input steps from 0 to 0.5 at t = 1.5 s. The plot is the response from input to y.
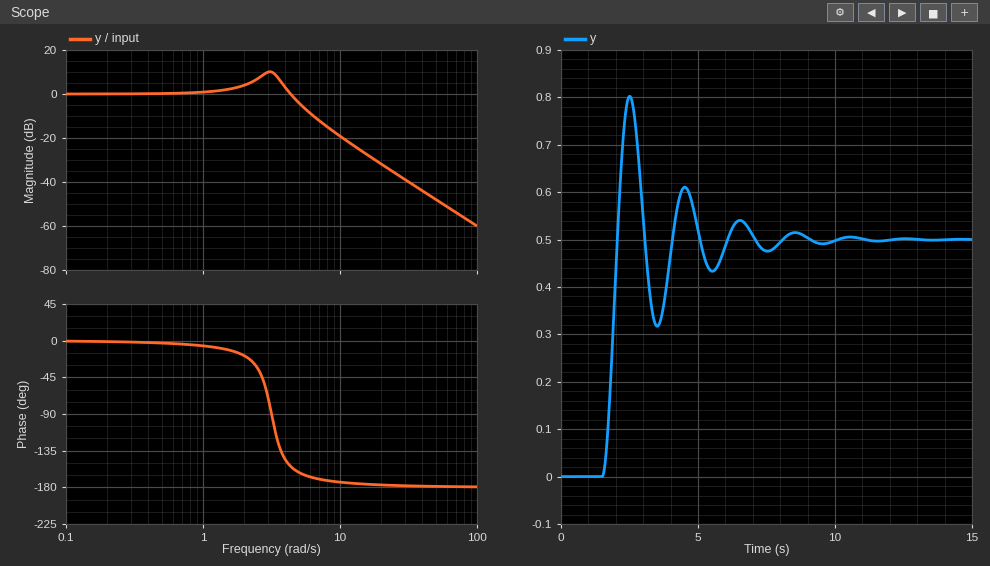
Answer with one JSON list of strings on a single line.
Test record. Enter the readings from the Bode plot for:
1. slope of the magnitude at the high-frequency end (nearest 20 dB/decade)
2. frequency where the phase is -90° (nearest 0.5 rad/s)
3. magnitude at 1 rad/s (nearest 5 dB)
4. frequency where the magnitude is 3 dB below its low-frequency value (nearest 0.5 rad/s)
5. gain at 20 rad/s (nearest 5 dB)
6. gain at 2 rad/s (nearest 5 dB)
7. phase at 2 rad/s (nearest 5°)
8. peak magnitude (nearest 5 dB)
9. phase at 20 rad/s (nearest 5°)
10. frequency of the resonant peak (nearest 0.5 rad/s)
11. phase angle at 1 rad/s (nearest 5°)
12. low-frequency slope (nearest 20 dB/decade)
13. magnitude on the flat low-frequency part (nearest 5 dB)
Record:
["-40 dB/decade", "3.0 rad/s", "0 dB", "5.0 rad/s", "-30 dB", "5 dB", "-20°", "10 dB", "-175°", "3.0 rad/s", "-5°", "0 dB/decade", "0 dB"]
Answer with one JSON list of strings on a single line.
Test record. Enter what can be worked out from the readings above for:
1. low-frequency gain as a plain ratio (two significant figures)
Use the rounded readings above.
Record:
["1.0"]
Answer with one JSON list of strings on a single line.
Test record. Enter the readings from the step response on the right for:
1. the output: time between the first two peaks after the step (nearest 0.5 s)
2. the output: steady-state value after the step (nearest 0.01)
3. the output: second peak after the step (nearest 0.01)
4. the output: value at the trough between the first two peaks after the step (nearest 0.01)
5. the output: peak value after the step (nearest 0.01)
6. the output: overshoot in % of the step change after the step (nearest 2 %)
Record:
["2.0 s", "0.50", "0.61", "0.32", "0.80", "60 %"]
